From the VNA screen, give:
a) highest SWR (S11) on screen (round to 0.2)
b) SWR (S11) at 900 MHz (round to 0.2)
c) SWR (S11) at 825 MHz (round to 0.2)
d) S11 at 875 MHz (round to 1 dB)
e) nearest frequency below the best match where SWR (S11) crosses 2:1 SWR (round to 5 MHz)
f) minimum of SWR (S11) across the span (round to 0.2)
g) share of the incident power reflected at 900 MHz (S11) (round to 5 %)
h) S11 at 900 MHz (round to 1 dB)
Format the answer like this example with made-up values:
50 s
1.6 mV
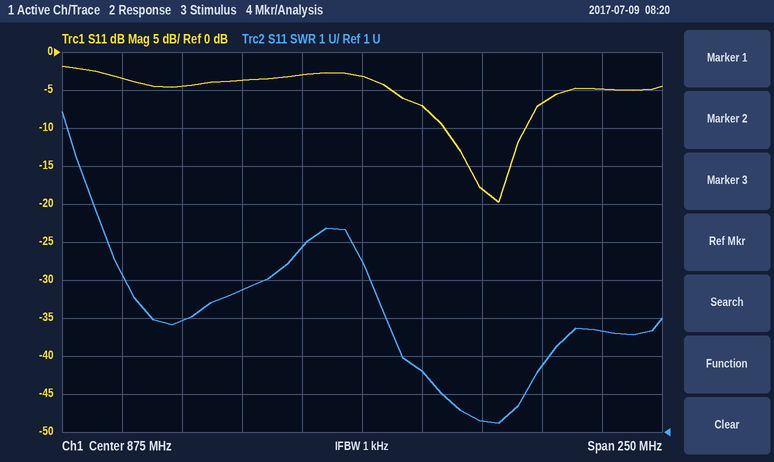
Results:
9.4
2.6
4.8
-3 dB
910 MHz
1.2
20 %
-7 dB
